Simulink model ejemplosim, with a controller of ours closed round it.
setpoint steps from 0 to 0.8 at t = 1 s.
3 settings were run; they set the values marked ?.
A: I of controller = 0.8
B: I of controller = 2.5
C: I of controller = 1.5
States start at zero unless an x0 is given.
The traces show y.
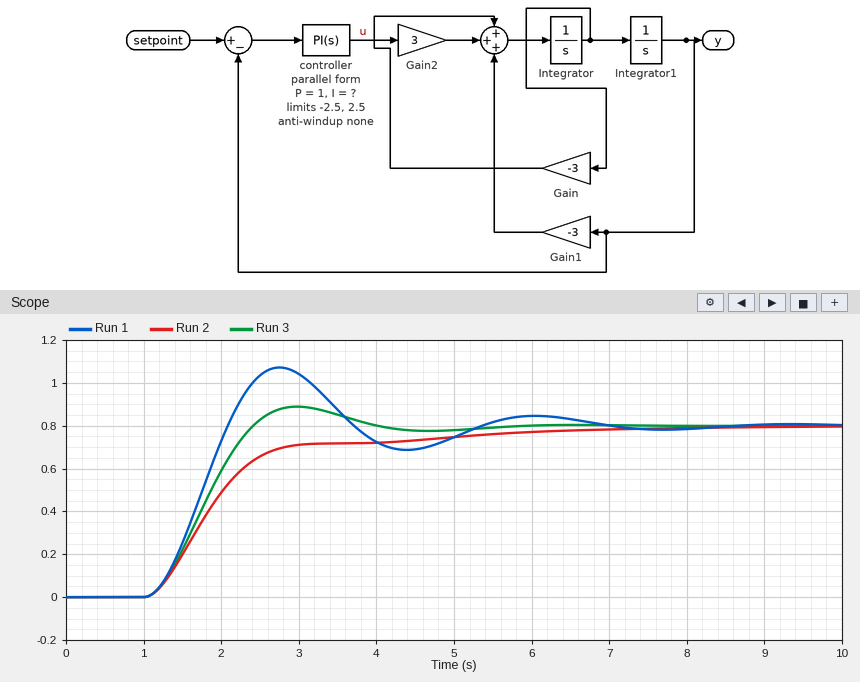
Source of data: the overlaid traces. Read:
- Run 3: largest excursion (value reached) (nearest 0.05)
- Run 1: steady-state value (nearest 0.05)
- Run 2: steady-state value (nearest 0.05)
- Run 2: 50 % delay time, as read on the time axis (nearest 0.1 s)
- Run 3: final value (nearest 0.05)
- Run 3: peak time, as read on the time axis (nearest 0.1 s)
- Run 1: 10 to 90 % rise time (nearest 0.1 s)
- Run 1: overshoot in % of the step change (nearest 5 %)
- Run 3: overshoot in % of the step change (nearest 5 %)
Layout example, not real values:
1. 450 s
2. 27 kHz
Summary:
1. 0.90
2. 0.80
3. 0.80
4. 1.8 s
5. 0.80
6. 3.0 s
7. 0.7 s
8. 35 %
9. 10 %
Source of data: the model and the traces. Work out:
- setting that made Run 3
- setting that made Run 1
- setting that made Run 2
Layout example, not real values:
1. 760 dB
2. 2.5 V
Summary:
1. C
2. B
3. A
